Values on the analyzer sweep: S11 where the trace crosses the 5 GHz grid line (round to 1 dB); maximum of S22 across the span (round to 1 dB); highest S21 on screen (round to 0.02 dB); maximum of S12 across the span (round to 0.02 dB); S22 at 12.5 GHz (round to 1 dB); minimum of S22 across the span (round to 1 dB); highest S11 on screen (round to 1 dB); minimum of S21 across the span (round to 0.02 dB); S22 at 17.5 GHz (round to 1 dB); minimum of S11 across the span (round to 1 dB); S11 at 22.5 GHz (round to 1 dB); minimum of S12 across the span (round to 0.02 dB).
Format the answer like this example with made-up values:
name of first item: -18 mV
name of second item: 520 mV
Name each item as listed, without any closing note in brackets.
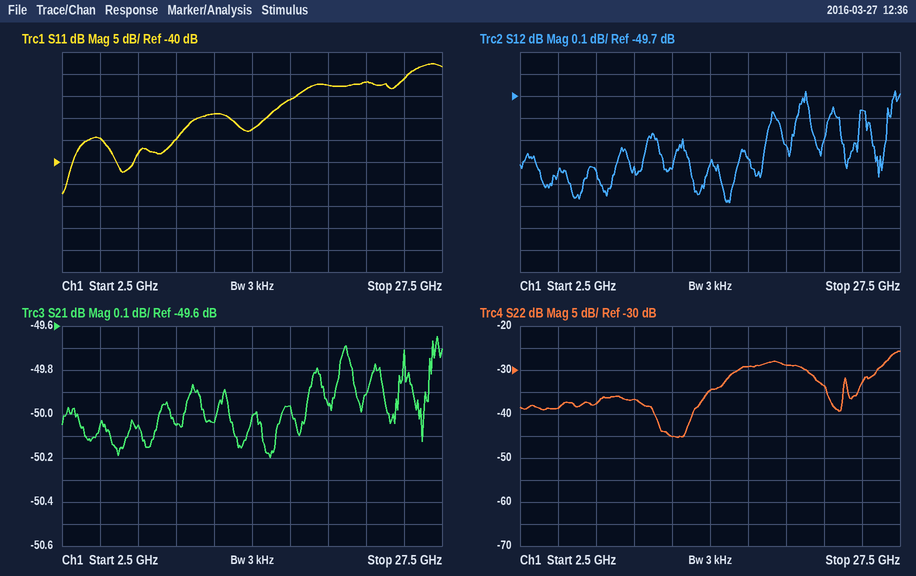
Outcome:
S11 where the trace crosses the 5 GHz grid line: -35 dB
maximum of S22 across the span: -26 dB
highest S21 on screen: -49.64 dB
maximum of S12 across the span: -49.68 dB
S22 at 12.5 GHz: -45 dB
minimum of S22 across the span: -45 dB
highest S11 on screen: -18 dB
minimum of S21 across the span: -50.20 dB
S22 at 17.5 GHz: -29 dB
minimum of S11 across the span: -47 dB
S11 at 22.5 GHz: -22 dB
minimum of S12 across the span: -50.18 dB
